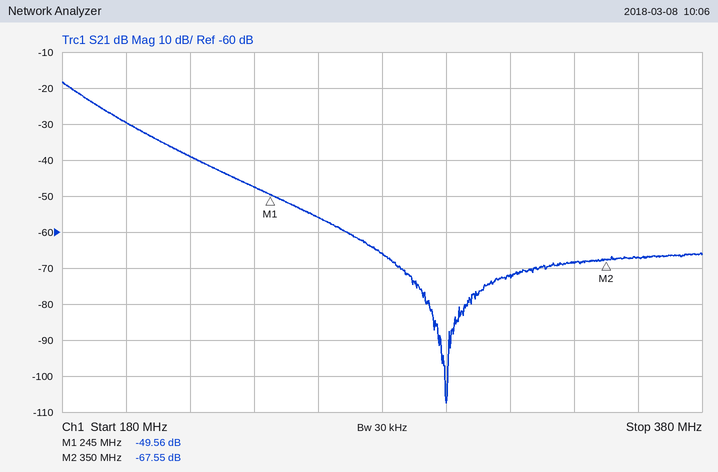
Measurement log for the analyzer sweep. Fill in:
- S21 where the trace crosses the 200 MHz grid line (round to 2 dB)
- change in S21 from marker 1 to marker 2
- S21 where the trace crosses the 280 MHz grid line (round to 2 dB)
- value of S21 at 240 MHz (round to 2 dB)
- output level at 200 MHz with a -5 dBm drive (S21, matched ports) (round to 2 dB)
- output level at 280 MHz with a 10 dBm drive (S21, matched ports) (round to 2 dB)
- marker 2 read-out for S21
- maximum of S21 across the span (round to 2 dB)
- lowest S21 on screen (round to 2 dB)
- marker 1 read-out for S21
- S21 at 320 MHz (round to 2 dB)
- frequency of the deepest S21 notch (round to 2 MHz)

-30 dB
-17.99 dB
-66 dB
-48 dB
-34 dBm
-56 dBm
-67.55 dB
-18 dB
-108 dB
-49.56 dB
-72 dB
300 MHz
